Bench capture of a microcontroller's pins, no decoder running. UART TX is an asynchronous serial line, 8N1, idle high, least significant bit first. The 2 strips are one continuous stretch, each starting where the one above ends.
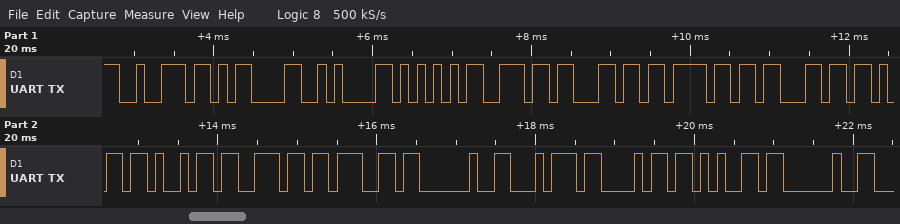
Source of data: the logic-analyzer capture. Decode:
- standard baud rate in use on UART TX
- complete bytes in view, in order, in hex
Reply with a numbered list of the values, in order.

1. 9600 baud
2. 72 0D 0A 55 6E 6C 6F 63 6B 69 6E 67 20 74 68 65 20
